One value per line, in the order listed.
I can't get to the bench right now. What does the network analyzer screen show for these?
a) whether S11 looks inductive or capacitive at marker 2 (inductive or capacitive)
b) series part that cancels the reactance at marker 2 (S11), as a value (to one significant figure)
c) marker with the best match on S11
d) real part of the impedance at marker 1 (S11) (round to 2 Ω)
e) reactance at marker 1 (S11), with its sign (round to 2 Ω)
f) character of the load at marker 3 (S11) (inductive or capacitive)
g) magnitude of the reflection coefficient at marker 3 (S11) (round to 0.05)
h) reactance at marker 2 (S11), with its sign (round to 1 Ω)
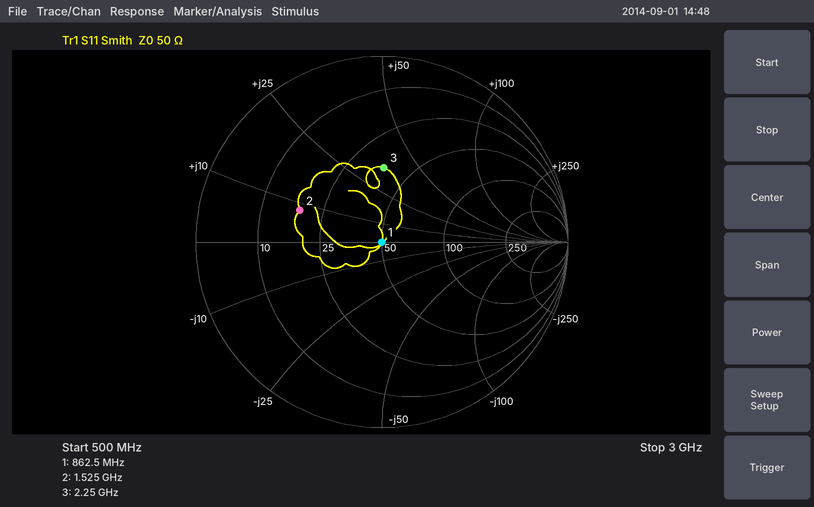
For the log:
inductive
10 pF
marker 1
50 Ω
0 Ω
inductive
0.40
+8 Ω
